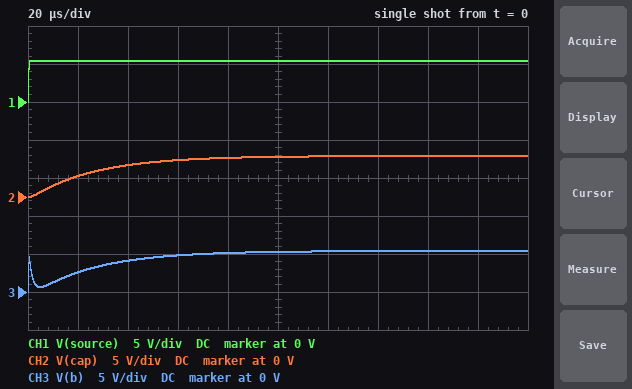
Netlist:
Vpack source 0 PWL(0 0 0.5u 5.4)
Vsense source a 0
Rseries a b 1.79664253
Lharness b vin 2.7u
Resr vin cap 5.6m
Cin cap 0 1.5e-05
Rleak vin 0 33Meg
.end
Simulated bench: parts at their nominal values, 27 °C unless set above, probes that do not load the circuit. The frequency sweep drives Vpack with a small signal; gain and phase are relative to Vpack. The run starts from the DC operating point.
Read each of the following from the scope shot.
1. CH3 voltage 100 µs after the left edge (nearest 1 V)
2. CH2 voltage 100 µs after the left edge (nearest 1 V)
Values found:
5 V
5 V
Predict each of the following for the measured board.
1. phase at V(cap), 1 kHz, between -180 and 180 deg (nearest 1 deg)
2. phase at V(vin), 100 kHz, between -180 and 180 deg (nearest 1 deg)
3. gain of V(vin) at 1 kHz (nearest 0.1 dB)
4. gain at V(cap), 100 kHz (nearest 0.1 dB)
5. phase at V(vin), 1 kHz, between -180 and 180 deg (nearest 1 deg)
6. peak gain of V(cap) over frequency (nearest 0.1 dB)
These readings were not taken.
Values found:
-10 deg
-128 deg
-0.1 dB
-27.1 dB
-10 deg
0 dB
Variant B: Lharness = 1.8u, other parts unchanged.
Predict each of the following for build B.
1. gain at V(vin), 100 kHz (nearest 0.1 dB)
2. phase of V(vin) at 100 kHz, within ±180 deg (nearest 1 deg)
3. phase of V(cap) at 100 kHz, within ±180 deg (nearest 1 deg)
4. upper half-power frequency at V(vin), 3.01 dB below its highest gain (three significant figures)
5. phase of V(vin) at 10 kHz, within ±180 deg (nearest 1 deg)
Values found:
-25.8 dB
-117 deg
-120 deg
6.11 kHz
-62 deg
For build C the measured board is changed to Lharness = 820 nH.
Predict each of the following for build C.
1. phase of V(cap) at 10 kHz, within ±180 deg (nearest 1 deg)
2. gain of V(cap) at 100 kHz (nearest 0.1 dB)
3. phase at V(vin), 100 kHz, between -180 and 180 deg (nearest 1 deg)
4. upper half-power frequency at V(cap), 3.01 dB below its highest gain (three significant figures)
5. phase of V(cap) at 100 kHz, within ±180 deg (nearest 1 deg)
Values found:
-61 deg
-24.8 dB
-100 deg
5.99 kHz
-103 deg
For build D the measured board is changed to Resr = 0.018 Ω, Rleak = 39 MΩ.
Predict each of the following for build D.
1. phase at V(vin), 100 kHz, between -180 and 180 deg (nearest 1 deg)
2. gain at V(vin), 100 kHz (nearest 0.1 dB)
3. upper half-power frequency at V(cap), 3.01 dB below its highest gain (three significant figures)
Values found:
-122 deg
-27.0 dB
6.18 kHz
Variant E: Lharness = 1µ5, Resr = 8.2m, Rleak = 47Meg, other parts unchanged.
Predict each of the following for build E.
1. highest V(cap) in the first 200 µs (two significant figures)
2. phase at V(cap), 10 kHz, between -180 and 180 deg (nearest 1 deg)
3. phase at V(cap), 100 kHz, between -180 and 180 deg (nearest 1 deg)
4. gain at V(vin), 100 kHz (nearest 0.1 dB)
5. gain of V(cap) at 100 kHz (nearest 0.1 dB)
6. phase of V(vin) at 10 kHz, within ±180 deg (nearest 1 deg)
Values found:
5.4 V
-62 deg
-115 deg
-25.4 dB
-25.5 dB
-61 deg
